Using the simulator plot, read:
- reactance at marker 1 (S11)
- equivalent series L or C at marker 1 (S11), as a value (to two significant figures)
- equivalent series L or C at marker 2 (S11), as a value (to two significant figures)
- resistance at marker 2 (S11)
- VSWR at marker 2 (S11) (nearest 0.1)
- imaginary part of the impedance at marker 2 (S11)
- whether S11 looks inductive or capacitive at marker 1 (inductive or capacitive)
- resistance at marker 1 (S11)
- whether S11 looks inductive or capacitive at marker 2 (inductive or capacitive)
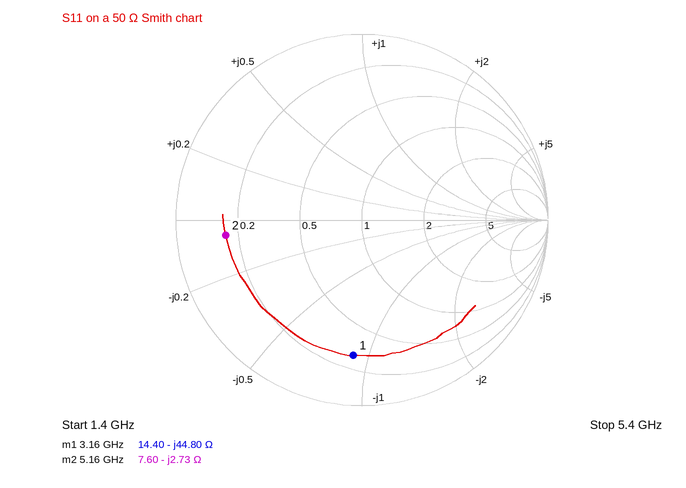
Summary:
-44.80 Ω
1.1 pF
11 pF
7.60 Ω
6.6
-2.73 Ω
capacitive
14.40 Ω
capacitive
